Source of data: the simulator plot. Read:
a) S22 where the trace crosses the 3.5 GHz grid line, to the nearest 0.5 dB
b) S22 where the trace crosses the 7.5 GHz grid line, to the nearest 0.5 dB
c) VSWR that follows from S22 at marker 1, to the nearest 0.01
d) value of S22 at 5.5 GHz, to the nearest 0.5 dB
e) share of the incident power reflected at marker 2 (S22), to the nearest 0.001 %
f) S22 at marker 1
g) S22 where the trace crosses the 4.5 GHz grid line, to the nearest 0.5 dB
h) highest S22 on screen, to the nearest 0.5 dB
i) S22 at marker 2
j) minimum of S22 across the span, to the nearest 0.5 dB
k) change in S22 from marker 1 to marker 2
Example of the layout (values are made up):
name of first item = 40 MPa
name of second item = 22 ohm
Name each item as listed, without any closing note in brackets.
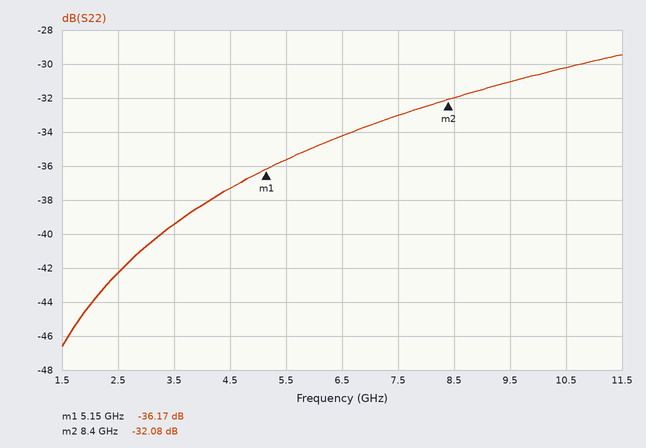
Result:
S22 where the trace crosses the 3.5 GHz grid line, to the nearest 0.5 dB = -39.5 dB
S22 where the trace crosses the 7.5 GHz grid line, to the nearest 0.5 dB = -33.0 dB
VSWR that follows from S22 at marker 1, to the nearest 0.01 = 1.03
value of S22 at 5.5 GHz, to the nearest 0.5 dB = -35.5 dB
share of the incident power reflected at marker 2 (S22), to the nearest 0.001 % = 0.062 %
S22 at marker 1 = -36.17 dB
S22 where the trace crosses the 4.5 GHz grid line, to the nearest 0.5 dB = -37.5 dB
highest S22 on screen, to the nearest 0.5 dB = -29.5 dB
S22 at marker 2 = -32.08 dB
minimum of S22 across the span, to the nearest 0.5 dB = -46.5 dB
change in S22 from marker 1 to marker 2 = 4.09 dB
